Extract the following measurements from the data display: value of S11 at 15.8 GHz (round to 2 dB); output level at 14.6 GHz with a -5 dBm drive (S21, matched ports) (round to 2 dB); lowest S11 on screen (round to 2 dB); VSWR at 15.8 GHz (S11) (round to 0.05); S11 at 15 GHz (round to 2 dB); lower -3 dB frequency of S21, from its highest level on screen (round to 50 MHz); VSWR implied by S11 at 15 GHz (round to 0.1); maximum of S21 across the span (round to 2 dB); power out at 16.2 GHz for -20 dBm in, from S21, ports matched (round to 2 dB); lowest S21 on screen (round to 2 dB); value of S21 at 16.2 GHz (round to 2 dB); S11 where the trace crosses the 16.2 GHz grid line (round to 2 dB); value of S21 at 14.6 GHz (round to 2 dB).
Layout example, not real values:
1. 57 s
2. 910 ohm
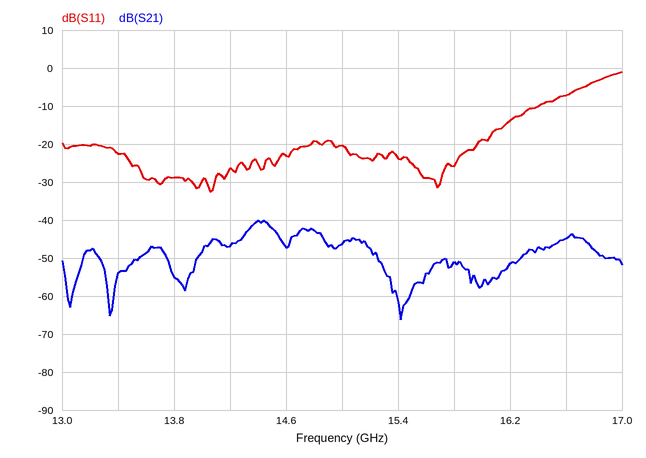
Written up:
1. -26 dB
2. -52 dBm
3. -32 dB
4. 1.10
5. -20 dB
6. 14.30 GHz
7. 1.2
8. -40 dB
9. -72 dBm
10. -66 dB
11. -52 dB
12. -14 dB
13. -48 dB
